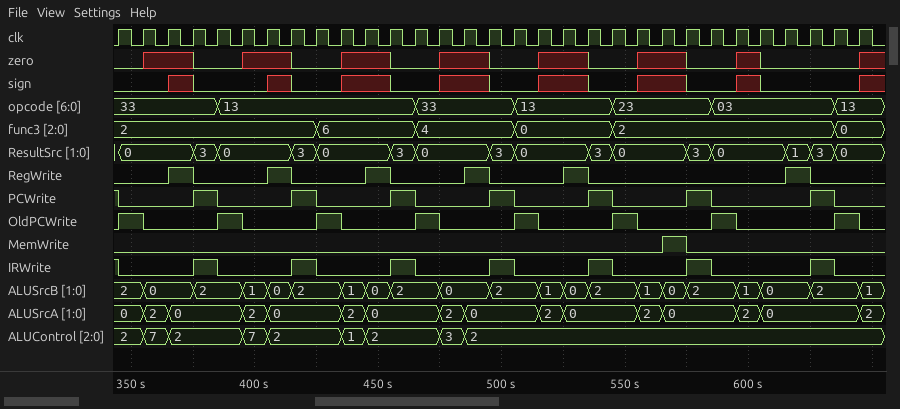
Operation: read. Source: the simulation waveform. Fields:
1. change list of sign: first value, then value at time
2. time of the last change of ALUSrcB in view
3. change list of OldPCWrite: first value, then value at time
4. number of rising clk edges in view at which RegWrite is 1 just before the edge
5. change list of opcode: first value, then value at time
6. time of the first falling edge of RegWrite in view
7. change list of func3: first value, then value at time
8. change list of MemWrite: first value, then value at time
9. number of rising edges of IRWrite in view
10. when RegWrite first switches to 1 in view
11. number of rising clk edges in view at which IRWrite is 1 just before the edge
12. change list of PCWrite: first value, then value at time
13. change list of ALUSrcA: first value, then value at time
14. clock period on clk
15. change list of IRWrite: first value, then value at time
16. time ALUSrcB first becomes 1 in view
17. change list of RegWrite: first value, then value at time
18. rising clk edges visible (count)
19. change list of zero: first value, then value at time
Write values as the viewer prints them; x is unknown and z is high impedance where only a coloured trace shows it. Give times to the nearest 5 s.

0, x at 365 s, 0 at 375 s, x at 405 s, 0 at 415 s, x at 435 s, 0 at 455 s, x at 475 s, 0 at 495 s, x at 515 s, 0 at 535 s, x at 555 s, 0 at 575 s, x at 595 s, 0 at 605 s, x at 645 s
645 s
0, 1 at 345 s, 0 at 355 s, 1 at 385 s, 0 at 395 s, 1 at 425 s, 0 at 435 s, 1 at 465 s, 0 at 475 s, 1 at 505 s, 0 at 515 s, 1 at 545 s, 0 at 555 s, 1 at 585 s, 0 at 595 s, 1 at 635 s, 0 at 645 s
6
33, 13 at 385 s, 33 at 465 s, 13 at 505 s, 23 at 545 s, 03 at 585 s, 13 at 635 s
375 s
2, 6 at 425 s, 4 at 465 s, 0 at 505 s, 2 at 545 s, 0 at 635 s
0, 1 at 565 s, 0 at 575 s
7
365 s
8
1, 0 at 345 s, 1 at 375 s, 0 at 385 s, 1 at 415 s, 0 at 425 s, 1 at 455 s, 0 at 465 s, 1 at 495 s, 0 at 505 s, 1 at 535 s, 0 at 545 s, 1 at 575 s, 0 at 585 s, 1 at 625 s, 0 at 635 s
0, 2 at 355 s, 0 at 365 s, 2 at 395 s, 0 at 405 s, 2 at 435 s, 0 at 445 s, 2 at 475 s, 0 at 485 s, 2 at 515 s, 0 at 525 s, 2 at 555 s, 0 at 565 s, 2 at 595 s, 0 at 605 s, 2 at 645 s
10 s
1, 0 at 345 s, 1 at 375 s, 0 at 385 s, 1 at 415 s, 0 at 425 s, 1 at 455 s, 0 at 465 s, 1 at 495 s, 0 at 505 s, 1 at 535 s, 0 at 545 s, 1 at 575 s, 0 at 585 s, 1 at 625 s, 0 at 635 s
395 s
0, 1 at 365 s, 0 at 375 s, 1 at 405 s, 0 at 415 s, 1 at 445 s, 0 at 455 s, 1 at 485 s, 0 at 495 s, 1 at 525 s, 0 at 535 s, 1 at 615 s, 0 at 625 s
31
0, x at 355 s, 0 at 375 s, x at 395 s, 0 at 415 s, x at 435 s, 0 at 455 s, x at 475 s, 0 at 495 s, x at 515 s, 0 at 535 s, x at 555 s, 0 at 575 s, x at 595 s, 0 at 605 s, x at 645 s
